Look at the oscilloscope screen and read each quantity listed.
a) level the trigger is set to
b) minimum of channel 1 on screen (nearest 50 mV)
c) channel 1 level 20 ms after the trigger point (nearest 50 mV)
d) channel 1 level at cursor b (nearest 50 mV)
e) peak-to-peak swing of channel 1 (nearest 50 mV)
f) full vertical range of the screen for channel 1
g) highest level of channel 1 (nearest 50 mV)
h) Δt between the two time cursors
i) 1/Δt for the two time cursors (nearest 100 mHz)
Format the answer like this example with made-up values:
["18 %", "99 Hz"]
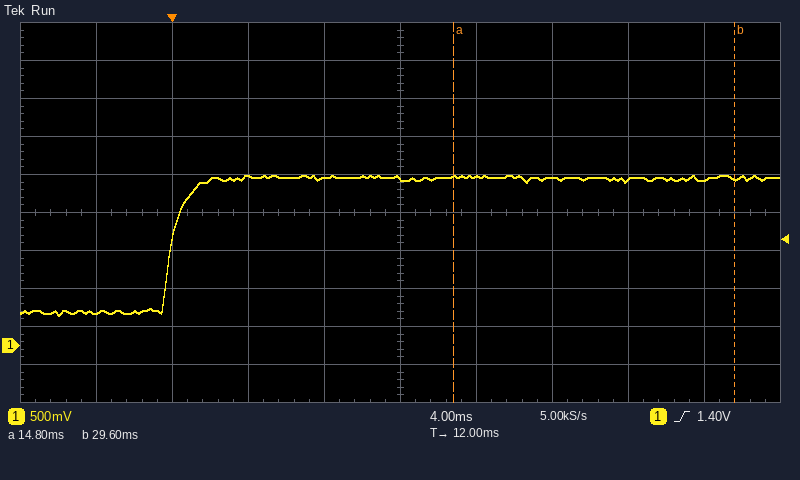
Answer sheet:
["1.40 V", "400 mV", "2.20 V", "2.20 V", "1.85 V", "5 V", "2.25 V", "14.8 ms", "67.6 Hz"]
